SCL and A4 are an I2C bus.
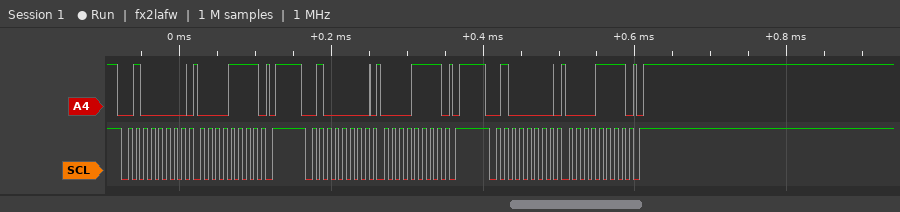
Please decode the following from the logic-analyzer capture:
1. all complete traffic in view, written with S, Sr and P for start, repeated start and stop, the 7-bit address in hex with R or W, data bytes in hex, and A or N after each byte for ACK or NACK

S 20W A 0F A P S 20W A 0F A P S 20W A 0F A P
